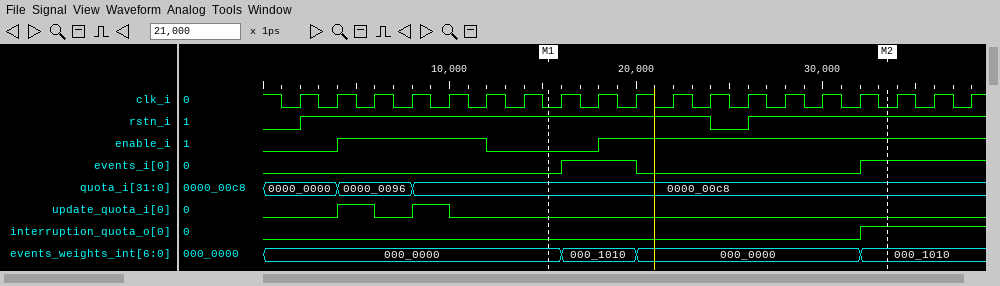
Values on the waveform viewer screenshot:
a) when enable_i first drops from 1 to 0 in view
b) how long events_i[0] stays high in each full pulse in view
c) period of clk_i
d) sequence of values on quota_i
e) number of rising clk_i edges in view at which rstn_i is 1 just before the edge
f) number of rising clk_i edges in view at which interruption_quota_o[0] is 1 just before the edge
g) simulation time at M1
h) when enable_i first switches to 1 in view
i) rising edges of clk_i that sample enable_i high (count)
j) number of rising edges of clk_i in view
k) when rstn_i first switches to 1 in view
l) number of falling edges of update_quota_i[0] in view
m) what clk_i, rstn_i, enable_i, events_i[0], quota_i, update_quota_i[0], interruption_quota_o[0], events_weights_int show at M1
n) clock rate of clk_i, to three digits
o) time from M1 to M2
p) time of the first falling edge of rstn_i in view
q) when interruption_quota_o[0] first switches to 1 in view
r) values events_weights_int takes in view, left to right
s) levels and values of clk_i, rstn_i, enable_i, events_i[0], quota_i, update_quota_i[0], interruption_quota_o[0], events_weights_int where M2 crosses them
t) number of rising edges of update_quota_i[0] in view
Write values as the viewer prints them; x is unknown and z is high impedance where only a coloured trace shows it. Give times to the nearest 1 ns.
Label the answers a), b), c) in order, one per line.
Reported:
a) 12 ns
b) 4 ns
c) 2 ns
d) 0000_0000, 0000_0096, 0000_00c8
e) 17
f) 3
g) 15 ns
h) 4 ns
i) 14
j) 19
k) 2 ns
l) 2
m) clk_i=0, rstn_i=1, enable_i=0, events_i[0]=0, quota_i=0000_00c8, update_quota_i[0]=0, interruption_quota_o[0]=0, events_weights_int=000_0000
n) 500 MHz
o) 18 ns
p) 24 ns
q) 32 ns
r) 000_0000, 000_1010, 000_0000, 000_1010
s) clk_i=0, rstn_i=1, enable_i=1, events_i[0]=1, quota_i=0000_00c8, update_quota_i[0]=0, interruption_quota_o[0]=1, events_weights_int=000_1010
t) 2
